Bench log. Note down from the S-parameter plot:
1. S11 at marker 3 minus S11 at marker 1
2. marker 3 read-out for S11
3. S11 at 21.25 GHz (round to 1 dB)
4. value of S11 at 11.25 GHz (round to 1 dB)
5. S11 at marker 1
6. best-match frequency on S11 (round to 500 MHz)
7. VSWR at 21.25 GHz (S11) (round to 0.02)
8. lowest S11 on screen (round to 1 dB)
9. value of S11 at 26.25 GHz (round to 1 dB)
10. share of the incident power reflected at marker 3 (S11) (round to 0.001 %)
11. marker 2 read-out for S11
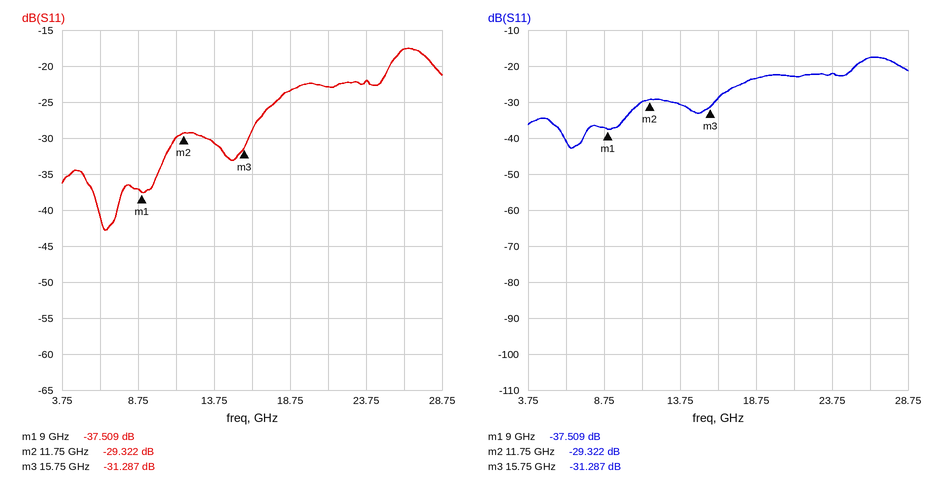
6.222 dB
-31.287 dB
-23 dB
-30 dB
-37.509 dB
6.5 GHz
1.16
-43 dB
-18 dB
0.074 %
-29.322 dB
